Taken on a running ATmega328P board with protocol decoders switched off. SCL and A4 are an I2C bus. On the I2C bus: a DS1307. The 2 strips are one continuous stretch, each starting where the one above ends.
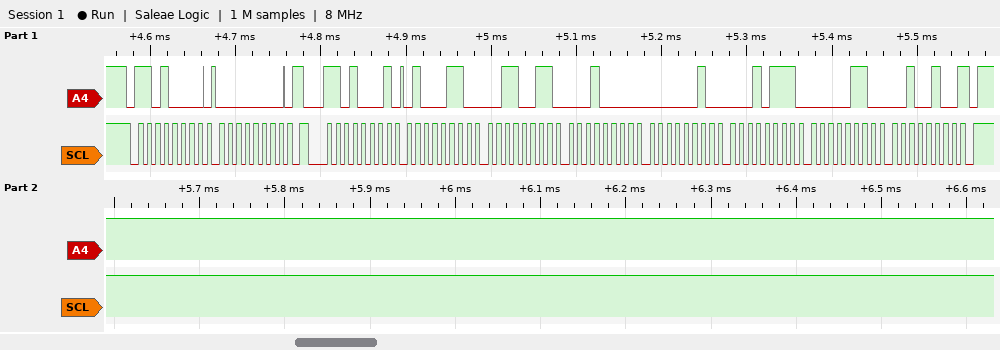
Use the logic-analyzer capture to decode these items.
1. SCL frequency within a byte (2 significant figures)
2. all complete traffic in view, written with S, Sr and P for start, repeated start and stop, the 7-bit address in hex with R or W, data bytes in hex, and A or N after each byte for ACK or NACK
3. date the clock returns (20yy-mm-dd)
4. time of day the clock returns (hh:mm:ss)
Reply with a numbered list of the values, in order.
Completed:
1. 100 kHz
2. S 68W A 00 A Sr 68R A 46 A 33 A 10 A 02 A 17 A 06 A 24 N P
3. 2024-06-17
4. 10:33:46
